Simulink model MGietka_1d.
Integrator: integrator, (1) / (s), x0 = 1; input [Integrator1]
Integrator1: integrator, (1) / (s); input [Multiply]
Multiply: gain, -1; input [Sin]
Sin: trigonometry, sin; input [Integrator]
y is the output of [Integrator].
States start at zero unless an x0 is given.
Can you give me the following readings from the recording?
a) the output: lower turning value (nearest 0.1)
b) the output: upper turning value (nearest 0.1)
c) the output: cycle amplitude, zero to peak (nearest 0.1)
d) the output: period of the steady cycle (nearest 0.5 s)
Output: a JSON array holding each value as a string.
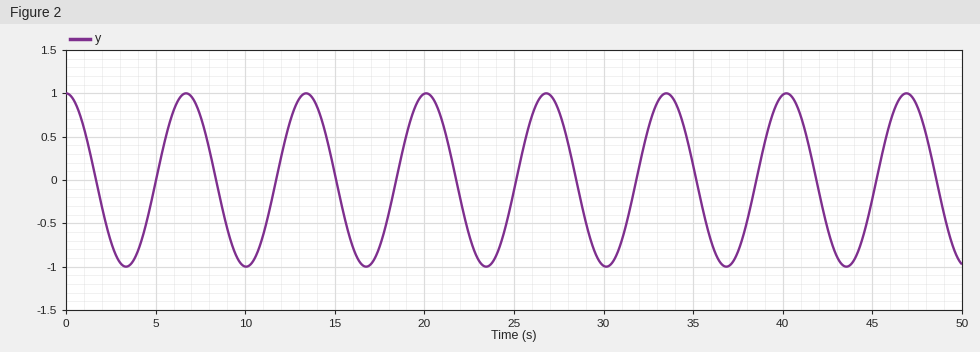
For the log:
["-1.0", "1.0", "1.0", "6.5 s"]
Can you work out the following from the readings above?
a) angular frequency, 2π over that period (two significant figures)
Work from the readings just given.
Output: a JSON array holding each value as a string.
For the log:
["0.97 rad/s"]
